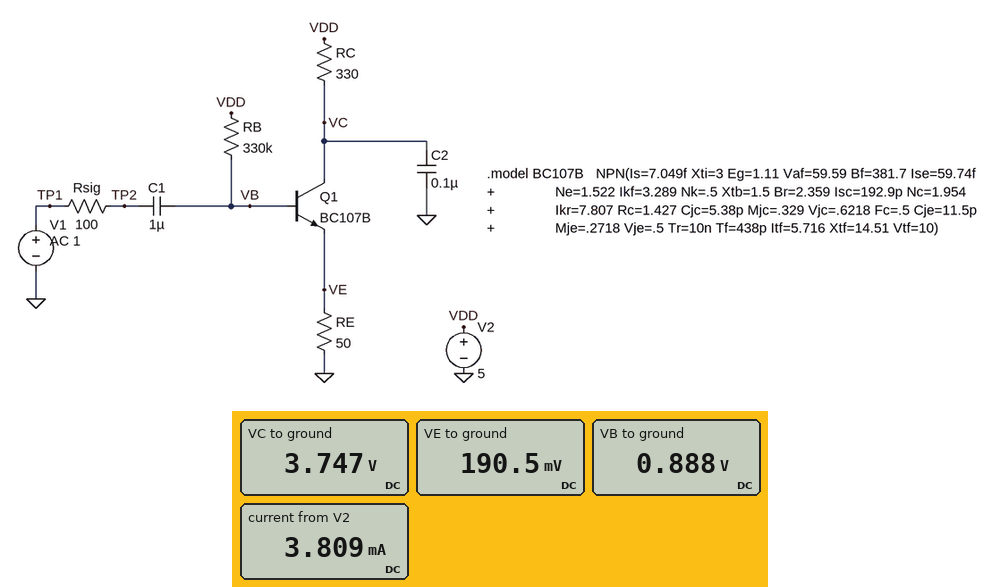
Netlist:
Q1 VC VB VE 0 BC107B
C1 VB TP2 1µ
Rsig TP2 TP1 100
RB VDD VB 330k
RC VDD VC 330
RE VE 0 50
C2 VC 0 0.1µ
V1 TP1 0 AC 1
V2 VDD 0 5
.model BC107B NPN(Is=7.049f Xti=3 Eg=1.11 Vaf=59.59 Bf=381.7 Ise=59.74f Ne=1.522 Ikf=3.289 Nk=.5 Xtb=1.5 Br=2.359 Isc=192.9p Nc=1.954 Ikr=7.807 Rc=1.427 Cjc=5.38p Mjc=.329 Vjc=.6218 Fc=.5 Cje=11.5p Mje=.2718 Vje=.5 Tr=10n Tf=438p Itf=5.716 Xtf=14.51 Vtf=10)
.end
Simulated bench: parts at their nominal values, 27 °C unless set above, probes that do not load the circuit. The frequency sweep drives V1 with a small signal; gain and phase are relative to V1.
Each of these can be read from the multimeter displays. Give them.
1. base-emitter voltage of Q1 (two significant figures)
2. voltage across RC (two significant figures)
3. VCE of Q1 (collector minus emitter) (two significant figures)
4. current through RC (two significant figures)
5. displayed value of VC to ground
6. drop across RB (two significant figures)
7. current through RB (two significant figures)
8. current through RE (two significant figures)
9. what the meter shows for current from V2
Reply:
700 mV
1.3 V
3.6 V
3.8 mA
3.747 V
4.1 V
12 µA
3.8 mA
3.809 mA
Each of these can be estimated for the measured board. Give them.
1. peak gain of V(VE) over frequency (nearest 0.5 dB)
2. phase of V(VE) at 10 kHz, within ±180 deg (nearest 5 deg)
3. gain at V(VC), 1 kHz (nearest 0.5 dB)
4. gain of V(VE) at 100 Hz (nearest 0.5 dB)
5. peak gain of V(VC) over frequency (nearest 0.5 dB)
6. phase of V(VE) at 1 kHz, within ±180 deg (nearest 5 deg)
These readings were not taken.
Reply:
-1.0 dB
0 deg
15.0 dB
-1.0 dB
15.0 dB
0 deg
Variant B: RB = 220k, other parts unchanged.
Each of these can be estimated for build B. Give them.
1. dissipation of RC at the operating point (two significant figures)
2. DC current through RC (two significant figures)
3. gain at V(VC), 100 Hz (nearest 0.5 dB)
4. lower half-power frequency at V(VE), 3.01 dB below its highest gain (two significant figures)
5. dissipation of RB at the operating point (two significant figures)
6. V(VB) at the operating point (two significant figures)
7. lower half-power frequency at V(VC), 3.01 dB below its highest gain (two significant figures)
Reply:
11 mW
5.7 mA
15.5 dB
9.7 Hz
73 µW
990 mV
9.6 Hz
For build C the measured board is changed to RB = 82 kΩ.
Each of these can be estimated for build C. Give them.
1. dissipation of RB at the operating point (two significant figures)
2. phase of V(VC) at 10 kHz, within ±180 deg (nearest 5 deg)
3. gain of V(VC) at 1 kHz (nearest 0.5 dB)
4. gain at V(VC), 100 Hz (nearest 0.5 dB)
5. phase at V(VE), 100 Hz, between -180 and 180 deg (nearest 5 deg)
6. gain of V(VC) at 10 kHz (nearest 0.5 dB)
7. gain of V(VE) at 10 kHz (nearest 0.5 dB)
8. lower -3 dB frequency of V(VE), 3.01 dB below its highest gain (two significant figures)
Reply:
160 µW
120 deg
15.0 dB
11.0 dB
50 deg
8.5 dB
-0.5 dB
130 Hz
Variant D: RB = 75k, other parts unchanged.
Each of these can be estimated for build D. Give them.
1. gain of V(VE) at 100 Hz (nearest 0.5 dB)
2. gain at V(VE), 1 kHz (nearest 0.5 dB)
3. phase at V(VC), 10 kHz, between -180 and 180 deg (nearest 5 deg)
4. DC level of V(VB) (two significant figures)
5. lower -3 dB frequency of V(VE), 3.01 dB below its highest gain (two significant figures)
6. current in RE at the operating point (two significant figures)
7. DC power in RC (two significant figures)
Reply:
-8.5 dB
-1.5 dB
120 deg
1.4 V
250 Hz
13 mA
52 mW
